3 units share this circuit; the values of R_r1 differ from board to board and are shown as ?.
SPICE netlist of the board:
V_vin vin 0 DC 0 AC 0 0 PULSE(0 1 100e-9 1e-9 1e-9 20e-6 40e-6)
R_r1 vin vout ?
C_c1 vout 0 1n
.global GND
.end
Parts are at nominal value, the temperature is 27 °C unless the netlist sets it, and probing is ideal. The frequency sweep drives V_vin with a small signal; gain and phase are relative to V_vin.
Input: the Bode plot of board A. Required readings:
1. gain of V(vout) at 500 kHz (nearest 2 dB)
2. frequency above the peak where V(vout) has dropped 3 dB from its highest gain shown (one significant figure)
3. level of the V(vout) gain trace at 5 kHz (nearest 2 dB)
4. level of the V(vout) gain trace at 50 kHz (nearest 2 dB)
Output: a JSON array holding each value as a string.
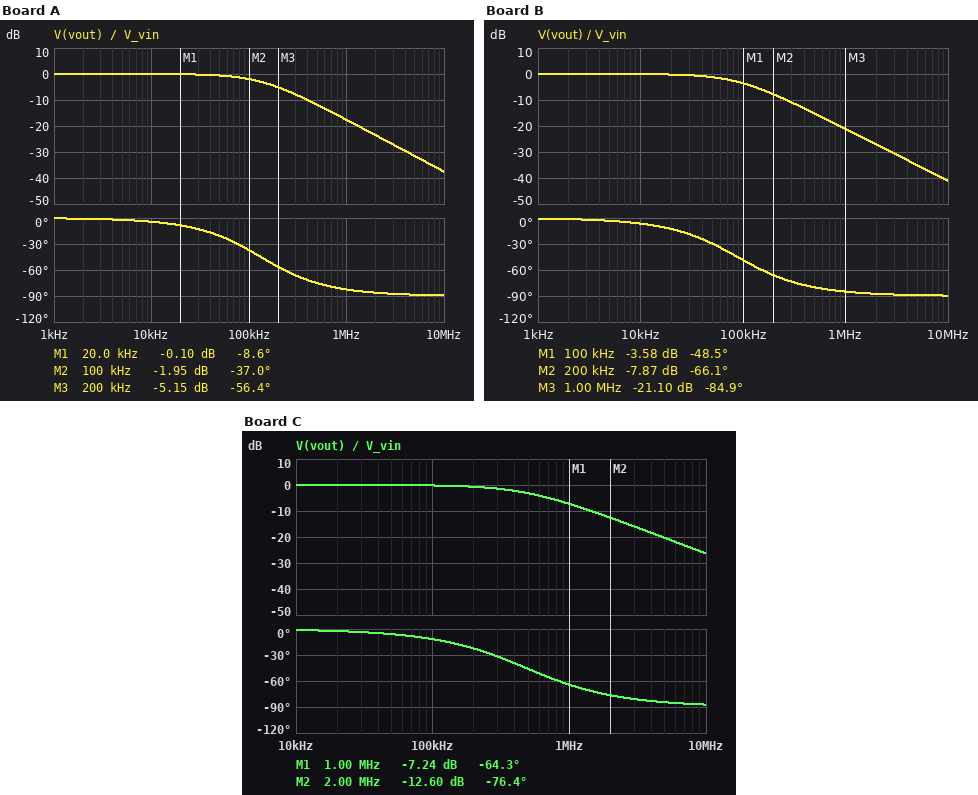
["-12 dB", "100 kHz", "0 dB", "0 dB"]
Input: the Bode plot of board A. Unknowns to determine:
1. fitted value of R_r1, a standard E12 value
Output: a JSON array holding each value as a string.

["1.2 kΩ"]
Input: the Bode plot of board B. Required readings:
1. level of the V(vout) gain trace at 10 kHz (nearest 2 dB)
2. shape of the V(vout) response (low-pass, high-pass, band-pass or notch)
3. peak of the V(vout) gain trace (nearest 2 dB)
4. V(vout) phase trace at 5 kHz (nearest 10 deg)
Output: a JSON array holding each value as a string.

["0 dB", "low-pass", "0 dB", "0 deg"]
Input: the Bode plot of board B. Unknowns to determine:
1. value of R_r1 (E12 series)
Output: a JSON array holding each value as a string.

["1.8 kΩ"]
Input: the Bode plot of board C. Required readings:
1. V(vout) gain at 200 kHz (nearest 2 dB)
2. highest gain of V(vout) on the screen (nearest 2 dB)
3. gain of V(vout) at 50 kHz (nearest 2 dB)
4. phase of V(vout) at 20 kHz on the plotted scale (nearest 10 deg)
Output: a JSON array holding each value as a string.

["0 dB", "0 dB", "0 dB", "0 deg"]
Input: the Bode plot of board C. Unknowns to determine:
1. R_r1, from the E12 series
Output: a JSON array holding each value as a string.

["330 Ω"]
